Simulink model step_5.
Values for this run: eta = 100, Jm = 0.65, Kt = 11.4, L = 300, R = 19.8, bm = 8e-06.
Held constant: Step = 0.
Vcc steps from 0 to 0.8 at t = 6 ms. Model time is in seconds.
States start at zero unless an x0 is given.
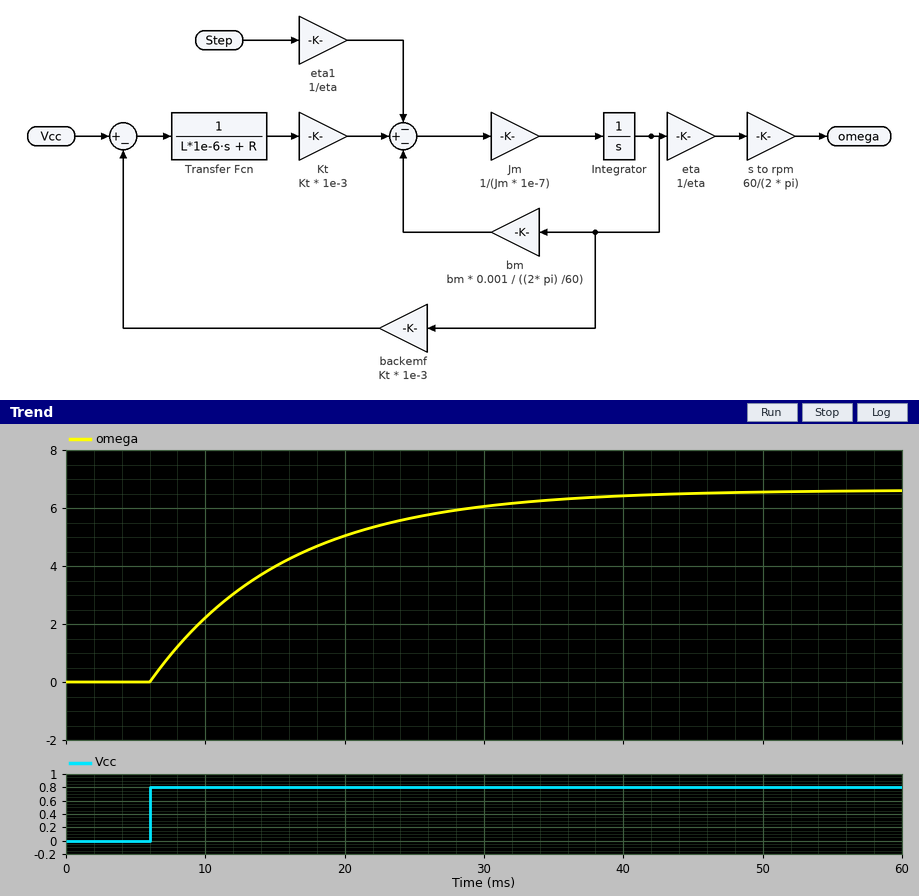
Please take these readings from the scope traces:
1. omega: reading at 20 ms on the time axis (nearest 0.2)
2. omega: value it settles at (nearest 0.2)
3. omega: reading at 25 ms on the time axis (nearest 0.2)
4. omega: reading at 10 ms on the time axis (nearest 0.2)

5.0
6.6
5.6
2.2
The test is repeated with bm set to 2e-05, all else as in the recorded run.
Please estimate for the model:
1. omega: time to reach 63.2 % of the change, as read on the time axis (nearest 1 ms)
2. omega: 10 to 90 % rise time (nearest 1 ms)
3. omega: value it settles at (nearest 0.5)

16 ms
21 ms
6.5
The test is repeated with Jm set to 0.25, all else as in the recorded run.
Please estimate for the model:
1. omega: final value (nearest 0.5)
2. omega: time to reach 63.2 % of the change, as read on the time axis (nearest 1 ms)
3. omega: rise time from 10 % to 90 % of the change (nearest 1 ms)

6.5
10 ms
8 ms
